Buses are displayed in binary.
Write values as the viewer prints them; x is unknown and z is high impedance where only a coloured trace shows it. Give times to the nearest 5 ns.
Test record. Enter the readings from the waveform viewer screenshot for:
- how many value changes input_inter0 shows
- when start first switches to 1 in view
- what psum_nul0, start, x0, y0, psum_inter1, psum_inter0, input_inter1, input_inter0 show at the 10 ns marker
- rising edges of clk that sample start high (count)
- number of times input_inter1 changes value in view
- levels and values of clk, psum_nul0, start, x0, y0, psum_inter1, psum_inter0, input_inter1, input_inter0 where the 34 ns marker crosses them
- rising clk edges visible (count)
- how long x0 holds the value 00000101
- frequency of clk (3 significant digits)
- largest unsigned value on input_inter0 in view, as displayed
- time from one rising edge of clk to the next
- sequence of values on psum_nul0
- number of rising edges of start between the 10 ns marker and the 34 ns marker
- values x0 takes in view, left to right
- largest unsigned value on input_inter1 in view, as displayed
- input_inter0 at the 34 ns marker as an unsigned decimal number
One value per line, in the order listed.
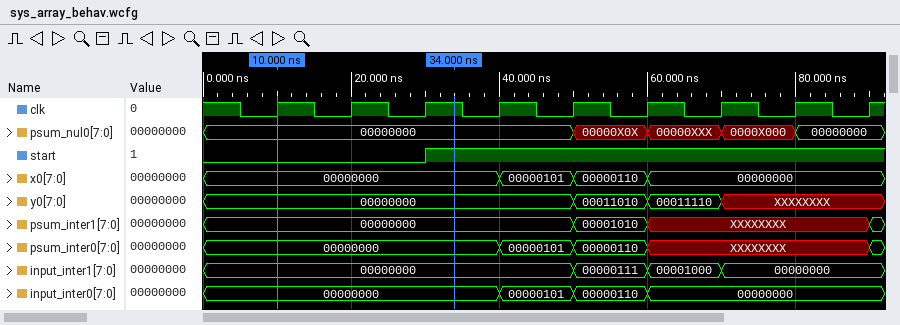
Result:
3
30 ns
psum_nul0=00000000, start=0, x0=00000000, y0=00000000, psum_inter1=00000000, psum_inter0=00000000, input_inter1=00000000, input_inter0=00000000
6
3
clk=1, psum_nul0=00000000, start=1, x0=00000000, y0=00000000, psum_inter1=00000000, psum_inter0=00000000, input_inter1=00000000, input_inter0=00000000
9
10 ns
100 MHz
00000110
10 ns
00000000, 00000X0X, 00000XXX, 0000X000, 00000000
1
00000000, 00000101, 00000110, 00000000
00001000
0
